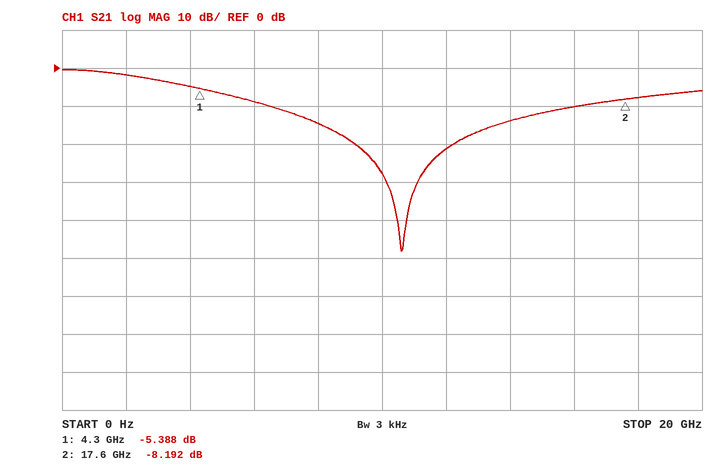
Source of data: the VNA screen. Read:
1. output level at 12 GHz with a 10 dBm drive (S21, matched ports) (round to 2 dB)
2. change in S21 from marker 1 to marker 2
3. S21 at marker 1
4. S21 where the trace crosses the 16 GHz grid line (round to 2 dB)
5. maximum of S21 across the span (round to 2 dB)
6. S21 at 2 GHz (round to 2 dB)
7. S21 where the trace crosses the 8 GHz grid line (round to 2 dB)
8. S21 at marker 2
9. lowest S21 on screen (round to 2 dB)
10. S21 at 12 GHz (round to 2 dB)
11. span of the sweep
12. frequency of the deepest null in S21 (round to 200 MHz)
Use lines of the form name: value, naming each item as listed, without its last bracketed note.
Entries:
output level at 12 GHz with a 10 dBm drive (S21, matched ports): -12 dBm
change in S21 from marker 1 to marker 2: -2.804 dB
S21 at marker 1: -5.388 dB
S21 where the trace crosses the 16 GHz grid line: -10 dB
maximum of S21 across the span: 0 dB
S21 at 2 GHz: -2 dB
S21 where the trace crosses the 8 GHz grid line: -14 dB
S21 at marker 2: -8.192 dB
lowest S21 on screen: -48 dB
S21 at 12 GHz: -22 dB
span of the sweep: 20 GHz
frequency of the deepest null in S21: 10.6 GHz
